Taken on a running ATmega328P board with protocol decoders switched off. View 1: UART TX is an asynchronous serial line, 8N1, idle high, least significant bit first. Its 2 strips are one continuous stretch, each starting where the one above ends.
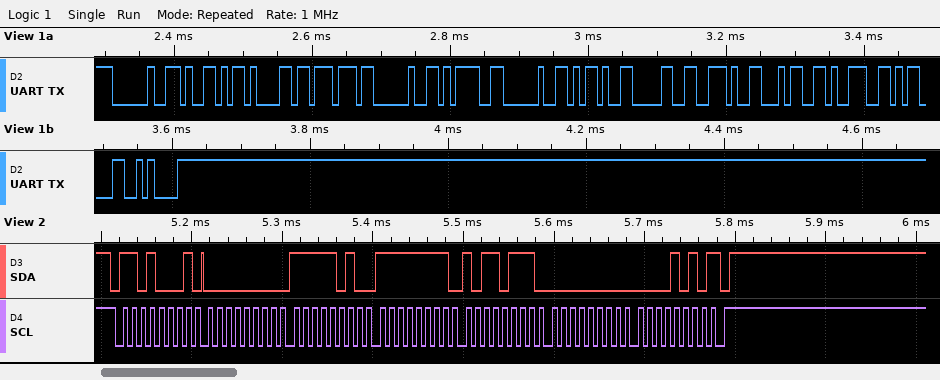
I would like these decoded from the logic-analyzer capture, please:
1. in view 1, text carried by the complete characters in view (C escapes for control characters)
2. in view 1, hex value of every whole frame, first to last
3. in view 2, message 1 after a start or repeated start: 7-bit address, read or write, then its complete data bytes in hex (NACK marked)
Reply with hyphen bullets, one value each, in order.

- " Yaw = -0.49\r\n"
- 20 59 61 77 20 3D 20 2D 30 2E 34 39 0D 0A
- 0x68 read: 00 FA FF B7 00 0A NACK
